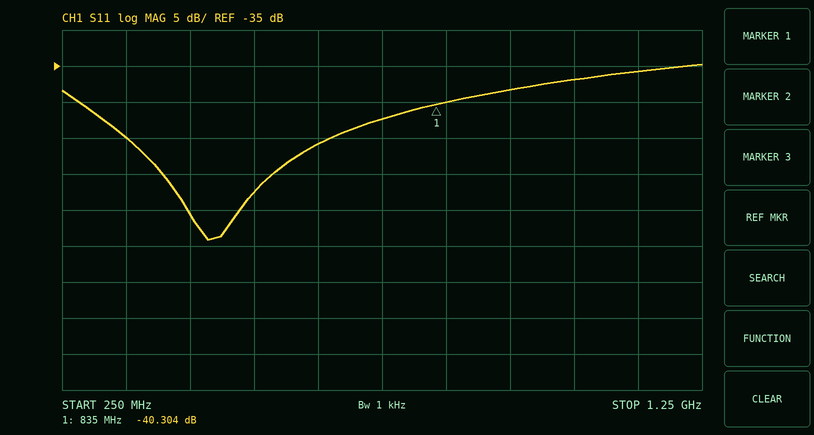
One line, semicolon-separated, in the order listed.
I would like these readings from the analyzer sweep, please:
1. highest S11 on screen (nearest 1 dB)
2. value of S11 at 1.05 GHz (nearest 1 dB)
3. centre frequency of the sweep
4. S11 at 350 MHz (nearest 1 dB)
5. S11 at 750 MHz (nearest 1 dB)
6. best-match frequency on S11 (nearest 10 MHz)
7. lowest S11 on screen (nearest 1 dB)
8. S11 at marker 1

-35 dB; -37 dB; 750 MHz; -45 dB; -42 dB; 480 MHz; -59 dB; -40.304 dB
